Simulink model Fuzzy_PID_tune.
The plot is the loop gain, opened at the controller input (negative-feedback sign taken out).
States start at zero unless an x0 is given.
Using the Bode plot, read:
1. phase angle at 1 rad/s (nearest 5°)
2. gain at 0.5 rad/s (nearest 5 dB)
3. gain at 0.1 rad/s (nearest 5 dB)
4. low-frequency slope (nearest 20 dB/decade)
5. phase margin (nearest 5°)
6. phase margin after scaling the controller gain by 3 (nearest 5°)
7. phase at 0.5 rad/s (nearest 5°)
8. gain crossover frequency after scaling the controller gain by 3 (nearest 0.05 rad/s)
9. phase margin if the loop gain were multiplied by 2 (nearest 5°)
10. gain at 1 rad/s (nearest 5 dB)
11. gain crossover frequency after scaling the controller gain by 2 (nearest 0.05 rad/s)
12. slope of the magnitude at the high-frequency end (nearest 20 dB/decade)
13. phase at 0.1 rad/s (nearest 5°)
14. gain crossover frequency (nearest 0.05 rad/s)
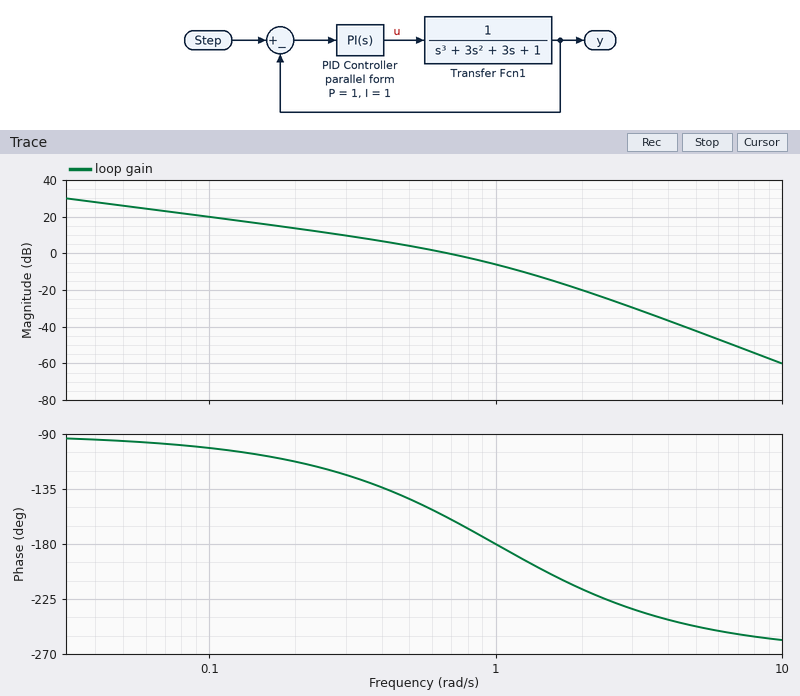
-180°
5 dB
20 dB
-20 dB/decade
20°
-10°
-145°
1.20 rad/s
0°
-5 dB
1.00 rad/s
-60 dB/decade
-100°
0.70 rad/s
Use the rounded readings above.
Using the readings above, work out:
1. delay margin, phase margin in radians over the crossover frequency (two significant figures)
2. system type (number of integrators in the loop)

0.50 s
1
